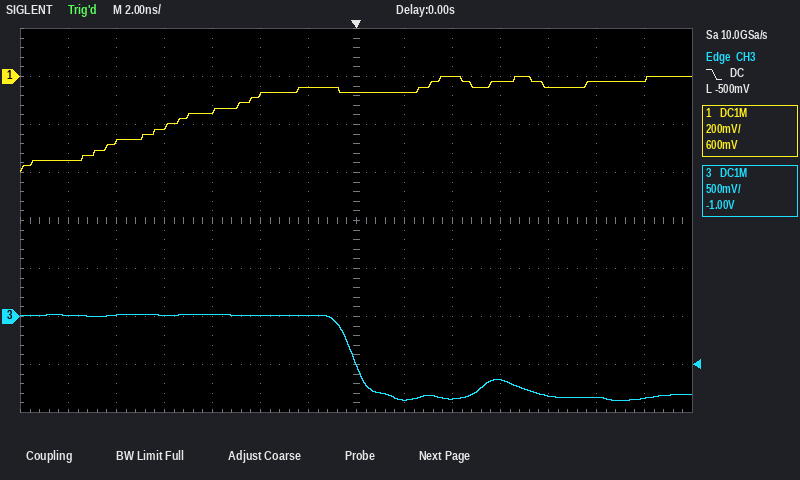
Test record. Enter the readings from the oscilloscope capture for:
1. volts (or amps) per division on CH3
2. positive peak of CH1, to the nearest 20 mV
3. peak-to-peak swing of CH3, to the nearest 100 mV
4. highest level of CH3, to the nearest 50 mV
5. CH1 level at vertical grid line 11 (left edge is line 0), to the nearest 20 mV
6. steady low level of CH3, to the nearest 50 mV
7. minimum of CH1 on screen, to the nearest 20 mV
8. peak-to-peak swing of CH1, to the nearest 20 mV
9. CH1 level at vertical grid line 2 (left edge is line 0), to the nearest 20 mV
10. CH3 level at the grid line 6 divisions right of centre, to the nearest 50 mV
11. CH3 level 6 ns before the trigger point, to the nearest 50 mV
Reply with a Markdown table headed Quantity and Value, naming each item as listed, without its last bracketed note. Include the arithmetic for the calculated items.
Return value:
| Quantity | Value |
|---|---|
| volts (or amps) per division on CH3 | 500 mV |
| positive peak of CH1, to the nearest 20 mV | 0 mV |
| peak-to-peak swing of CH3, to the nearest 100 mV | 900 mV |
| highest level of CH3, to the nearest 50 mV | 0 mV |
| CH1 level at vertical grid line 11 (left edge is line 0), to the nearest 20 mV | -40 mV |
| steady low level of CH3, to the nearest 50 mV | -850 mV |
| minimum of CH1 on screen, to the nearest 20 mV | -400 mV |
| peak-to-peak swing of CH1, to the nearest 20 mV | 0 mV − (-400 mV) = 400 mV |
| CH1 level at vertical grid line 2 (left edge is line 0), to the nearest 20 mV | -280 mV |
| CH3 level at the grid line 6 divisions right of centre, to the nearest 50 mV | -850 mV |
| CH3 level 6 ns before the trigger point, to the nearest 50 mV | 0 mV |
